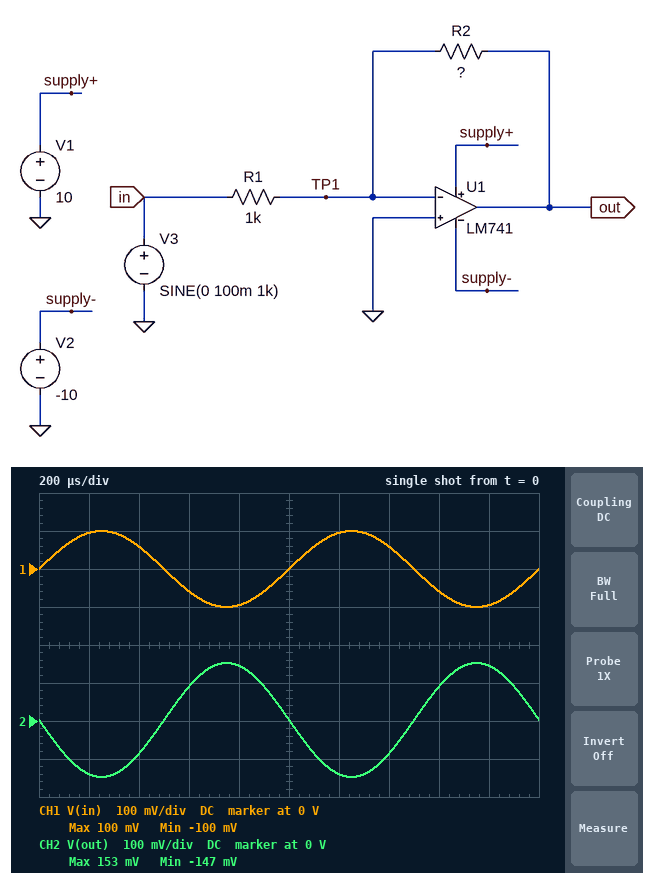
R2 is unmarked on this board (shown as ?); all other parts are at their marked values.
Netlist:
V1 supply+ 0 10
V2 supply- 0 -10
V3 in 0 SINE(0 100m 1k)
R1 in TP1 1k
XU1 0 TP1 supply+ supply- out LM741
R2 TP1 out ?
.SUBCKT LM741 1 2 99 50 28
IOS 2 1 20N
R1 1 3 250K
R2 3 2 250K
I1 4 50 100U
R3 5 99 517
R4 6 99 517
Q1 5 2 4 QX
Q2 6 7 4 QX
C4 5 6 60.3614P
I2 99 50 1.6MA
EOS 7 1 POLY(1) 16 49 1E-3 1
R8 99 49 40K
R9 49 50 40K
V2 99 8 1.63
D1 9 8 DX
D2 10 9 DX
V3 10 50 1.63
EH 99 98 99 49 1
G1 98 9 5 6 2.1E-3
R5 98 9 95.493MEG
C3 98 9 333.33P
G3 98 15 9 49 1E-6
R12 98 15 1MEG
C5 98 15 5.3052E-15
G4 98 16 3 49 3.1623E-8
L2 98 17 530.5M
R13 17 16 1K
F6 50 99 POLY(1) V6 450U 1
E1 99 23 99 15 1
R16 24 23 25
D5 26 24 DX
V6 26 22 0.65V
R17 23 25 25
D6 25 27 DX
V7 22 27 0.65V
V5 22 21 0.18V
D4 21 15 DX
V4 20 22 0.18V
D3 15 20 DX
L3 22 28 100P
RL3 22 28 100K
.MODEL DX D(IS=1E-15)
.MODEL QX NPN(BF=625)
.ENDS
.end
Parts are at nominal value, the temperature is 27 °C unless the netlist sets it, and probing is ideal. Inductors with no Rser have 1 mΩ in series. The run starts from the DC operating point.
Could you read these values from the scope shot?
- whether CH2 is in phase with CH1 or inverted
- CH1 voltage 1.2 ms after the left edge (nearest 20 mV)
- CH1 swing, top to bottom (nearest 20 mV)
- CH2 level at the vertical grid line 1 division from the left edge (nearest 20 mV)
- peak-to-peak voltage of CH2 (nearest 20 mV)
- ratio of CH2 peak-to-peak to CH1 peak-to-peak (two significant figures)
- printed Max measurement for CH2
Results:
inverted
100 mV
200 mV
-140 mV
300 mV
1.5
153 mV
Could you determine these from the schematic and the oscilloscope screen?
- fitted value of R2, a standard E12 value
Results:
1.5 kΩ
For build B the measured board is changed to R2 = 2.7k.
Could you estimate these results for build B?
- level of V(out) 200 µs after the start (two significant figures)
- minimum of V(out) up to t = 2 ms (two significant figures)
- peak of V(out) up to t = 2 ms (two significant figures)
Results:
-250 mV
-270 mV
270 mV
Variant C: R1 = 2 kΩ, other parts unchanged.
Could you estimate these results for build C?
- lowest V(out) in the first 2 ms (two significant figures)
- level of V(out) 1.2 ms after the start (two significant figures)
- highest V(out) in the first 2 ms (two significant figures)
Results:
-73 mV
-69 mV
77 mV
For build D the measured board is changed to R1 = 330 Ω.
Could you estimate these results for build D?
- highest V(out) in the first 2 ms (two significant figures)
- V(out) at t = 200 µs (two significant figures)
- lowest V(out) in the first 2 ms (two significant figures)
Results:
460 mV
-430 mV
-450 mV
